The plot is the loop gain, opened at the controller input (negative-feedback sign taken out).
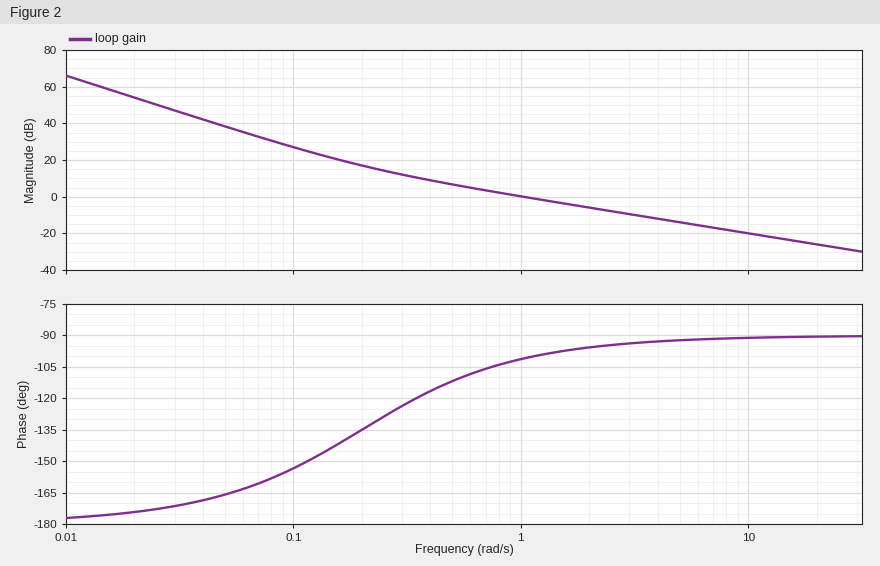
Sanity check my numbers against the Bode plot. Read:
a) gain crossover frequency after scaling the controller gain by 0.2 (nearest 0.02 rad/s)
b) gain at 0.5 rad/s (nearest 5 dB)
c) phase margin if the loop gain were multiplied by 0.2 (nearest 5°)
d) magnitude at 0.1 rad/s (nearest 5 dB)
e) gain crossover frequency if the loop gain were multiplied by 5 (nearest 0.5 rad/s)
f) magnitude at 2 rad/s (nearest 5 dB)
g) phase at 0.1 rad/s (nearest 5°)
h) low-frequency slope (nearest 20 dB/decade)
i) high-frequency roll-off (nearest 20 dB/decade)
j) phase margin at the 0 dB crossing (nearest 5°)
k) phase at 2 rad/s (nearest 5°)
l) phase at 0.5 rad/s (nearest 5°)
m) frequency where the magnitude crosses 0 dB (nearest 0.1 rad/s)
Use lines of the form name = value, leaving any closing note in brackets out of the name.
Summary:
gain crossover frequency after scaling the controller gain by 0.2 = 0.26 rad/s
gain at 0.5 rad/s = 5 dB
phase margin if the loop gain were multiplied by 0.2 = 50°
magnitude at 0.1 rad/s = 25 dB
gain crossover frequency if the loop gain were multiplied by 5 = 5.0 rad/s
magnitude at 2 rad/s = -5 dB
phase at 0.1 rad/s = -155°
low-frequency slope = -40 dB/decade
high-frequency roll-off = -20 dB/decade
phase margin at the 0 dB crossing = 80°
phase at 2 rad/s = -95°
phase at 0.5 rad/s = -110°
frequency where the magnitude crosses 0 dB = 1.0 rad/s
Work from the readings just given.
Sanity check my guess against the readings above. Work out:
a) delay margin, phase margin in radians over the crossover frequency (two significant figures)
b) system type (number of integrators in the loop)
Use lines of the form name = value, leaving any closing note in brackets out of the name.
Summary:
delay margin, phase margin in radians over the crossover frequency = 1.4 s
system type = 2
